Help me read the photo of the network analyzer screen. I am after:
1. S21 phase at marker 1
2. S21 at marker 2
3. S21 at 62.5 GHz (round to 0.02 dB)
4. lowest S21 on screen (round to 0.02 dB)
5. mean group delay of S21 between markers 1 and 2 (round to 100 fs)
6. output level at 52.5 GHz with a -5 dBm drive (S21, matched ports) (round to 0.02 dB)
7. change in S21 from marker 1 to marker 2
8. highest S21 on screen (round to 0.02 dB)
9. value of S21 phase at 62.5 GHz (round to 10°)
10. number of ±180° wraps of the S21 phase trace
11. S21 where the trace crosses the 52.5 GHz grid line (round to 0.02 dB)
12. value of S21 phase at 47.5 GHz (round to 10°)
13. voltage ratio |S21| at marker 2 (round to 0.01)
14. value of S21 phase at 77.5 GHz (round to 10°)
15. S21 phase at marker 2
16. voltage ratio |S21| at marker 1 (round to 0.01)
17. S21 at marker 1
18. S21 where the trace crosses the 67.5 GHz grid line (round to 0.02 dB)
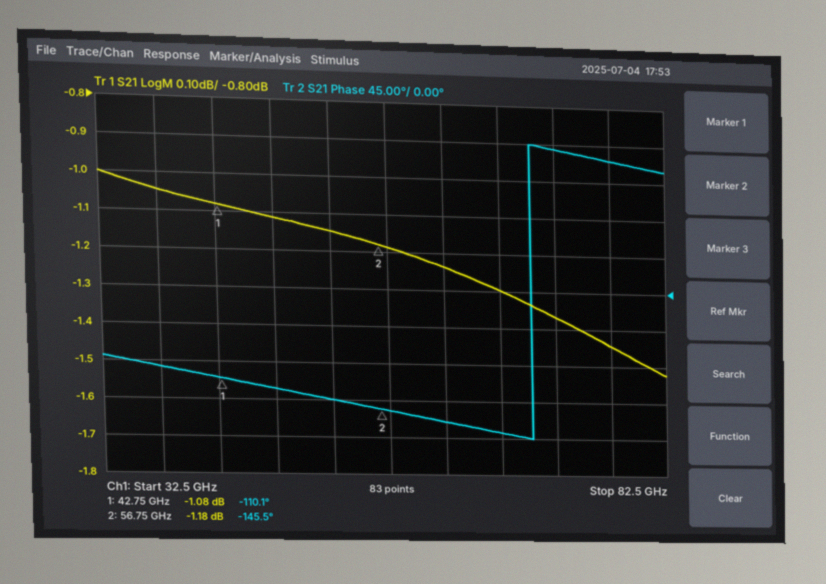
-110.1°
-1.18 dB
-1.24 dB
-1.52 dB
7.0 ps
-6.14 dBm
-0.10 dB
-1.00 dB
-160°
1
-1.14 dB
-120°
0.87
160°
-145.5°
0.88
-1.08 dB
-1.30 dB
